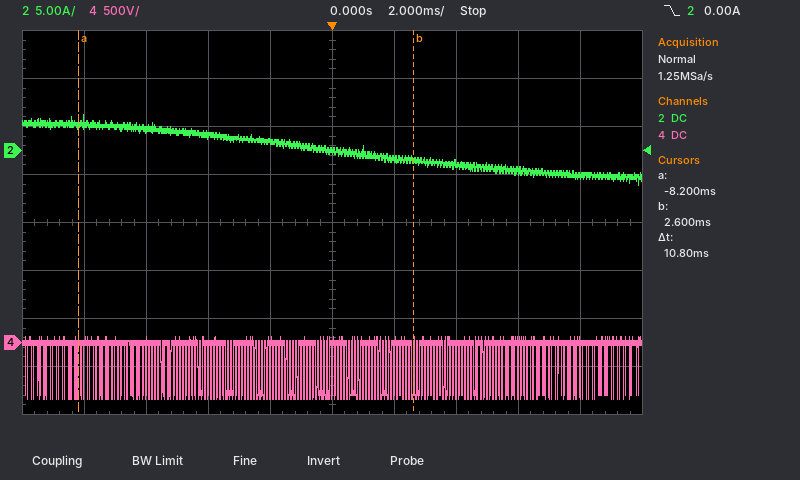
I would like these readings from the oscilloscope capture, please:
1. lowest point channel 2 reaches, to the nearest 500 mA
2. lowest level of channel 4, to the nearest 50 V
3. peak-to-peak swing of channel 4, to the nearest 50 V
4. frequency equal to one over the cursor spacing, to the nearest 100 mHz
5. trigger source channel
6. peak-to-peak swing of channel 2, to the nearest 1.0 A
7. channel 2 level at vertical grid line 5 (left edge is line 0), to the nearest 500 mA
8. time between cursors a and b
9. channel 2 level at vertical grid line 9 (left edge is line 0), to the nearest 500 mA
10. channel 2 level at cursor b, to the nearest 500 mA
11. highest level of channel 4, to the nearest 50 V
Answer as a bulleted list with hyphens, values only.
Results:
- -3.5 A
- -600 V
- 650 V
- 92.6 Hz
- channel 2
- 7.0 A
- 0.0 A
- 10.8 ms
- -2.5 A
- -1.0 A
- 50 V
